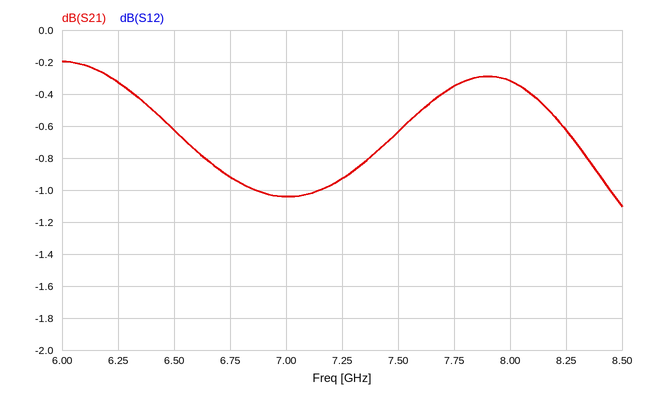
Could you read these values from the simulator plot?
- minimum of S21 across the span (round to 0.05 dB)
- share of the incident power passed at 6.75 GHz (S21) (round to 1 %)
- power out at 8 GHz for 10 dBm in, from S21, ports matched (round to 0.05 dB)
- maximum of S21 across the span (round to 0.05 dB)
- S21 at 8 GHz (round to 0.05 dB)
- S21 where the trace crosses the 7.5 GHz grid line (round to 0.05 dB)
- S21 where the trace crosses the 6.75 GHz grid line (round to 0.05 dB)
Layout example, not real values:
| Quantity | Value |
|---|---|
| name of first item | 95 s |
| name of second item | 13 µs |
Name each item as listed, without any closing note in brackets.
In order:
| Quantity | Value |
|---|---|
| minimum of S21 across the span | -1.10 dB |
| share of the incident power passed at 6.75 GHz (S21) | 81 % |
| power out at 8 GHz for 10 dBm in, from S21, ports matched | 9.70 dBm |
| maximum of S21 across the span | -0.20 dB |
| S21 at 8 GHz | -0.30 dB |
| S21 where the trace crosses the 7.5 GHz grid line | -0.65 dB |
| S21 where the trace crosses the 6.75 GHz grid line | -0.90 dB |
